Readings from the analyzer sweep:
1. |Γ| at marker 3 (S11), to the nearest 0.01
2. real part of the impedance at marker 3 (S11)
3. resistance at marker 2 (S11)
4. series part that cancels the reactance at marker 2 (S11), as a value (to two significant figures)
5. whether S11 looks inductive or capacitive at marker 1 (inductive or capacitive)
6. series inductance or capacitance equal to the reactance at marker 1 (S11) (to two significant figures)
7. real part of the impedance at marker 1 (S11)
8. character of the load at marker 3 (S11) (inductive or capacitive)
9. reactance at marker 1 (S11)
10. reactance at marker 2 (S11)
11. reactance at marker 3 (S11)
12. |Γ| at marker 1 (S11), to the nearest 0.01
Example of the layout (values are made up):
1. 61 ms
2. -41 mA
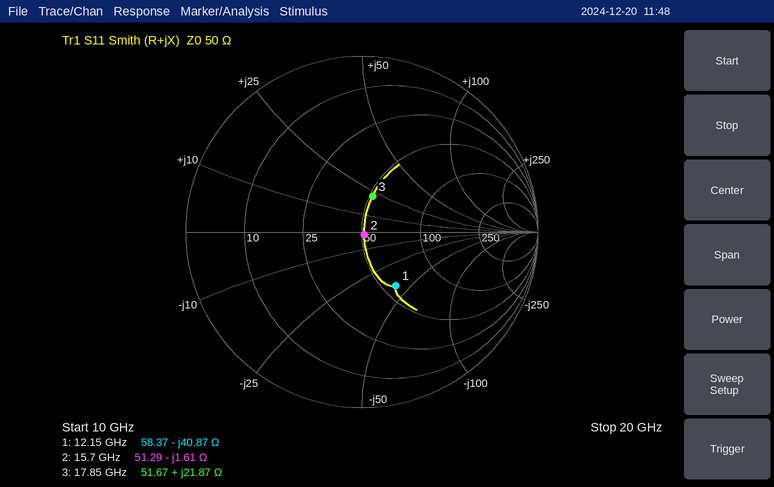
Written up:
1. 0.21
2. 51.67 Ω
3. 51.29 Ω
4. 16 pH
5. capacitive
6. 320 fF
7. 58.37 Ω
8. inductive
9. -40.87 Ω
10. -1.61 Ω
11. +21.87 Ω
12. 0.36
